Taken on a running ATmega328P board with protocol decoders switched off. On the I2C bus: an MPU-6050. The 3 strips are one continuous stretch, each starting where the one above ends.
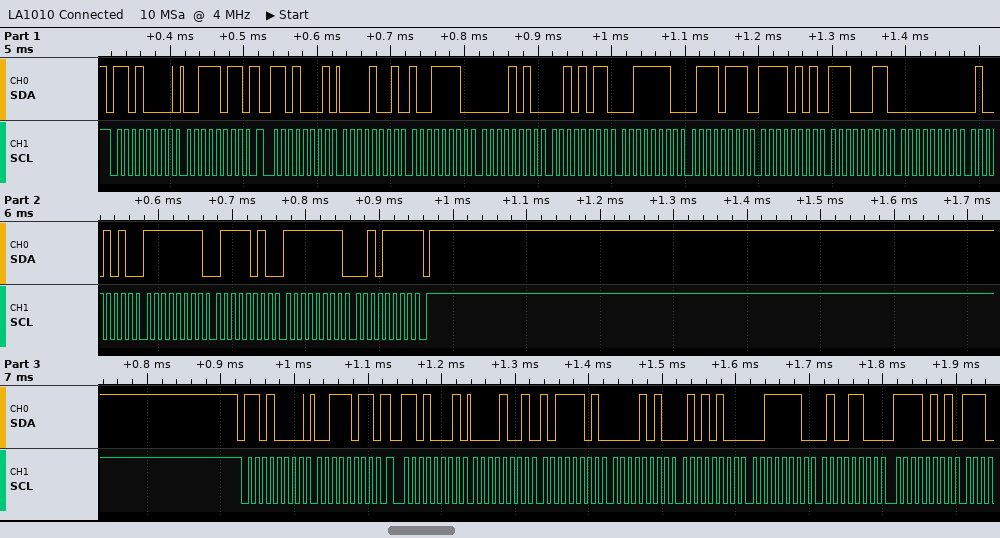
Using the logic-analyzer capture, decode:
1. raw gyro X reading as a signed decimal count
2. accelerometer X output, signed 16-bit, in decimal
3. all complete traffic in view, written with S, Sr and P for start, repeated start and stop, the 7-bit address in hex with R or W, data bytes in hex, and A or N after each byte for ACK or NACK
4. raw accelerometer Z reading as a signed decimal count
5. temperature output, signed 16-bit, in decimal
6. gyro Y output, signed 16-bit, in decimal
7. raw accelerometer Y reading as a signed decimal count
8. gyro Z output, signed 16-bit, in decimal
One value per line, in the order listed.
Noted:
74
2462
S 68W A 3B A Sr 68R A 09 A 9E A 0A A 2B A 3E A 77 A F5 A E3 A 00 A 4A A FF A 7A A FF A 2F N P S 68W A 3B A Sr 68R A 09 A BD A 0A A 54 A 3E A 4C A F5 A
15991
-2589
-134
2603
-209
